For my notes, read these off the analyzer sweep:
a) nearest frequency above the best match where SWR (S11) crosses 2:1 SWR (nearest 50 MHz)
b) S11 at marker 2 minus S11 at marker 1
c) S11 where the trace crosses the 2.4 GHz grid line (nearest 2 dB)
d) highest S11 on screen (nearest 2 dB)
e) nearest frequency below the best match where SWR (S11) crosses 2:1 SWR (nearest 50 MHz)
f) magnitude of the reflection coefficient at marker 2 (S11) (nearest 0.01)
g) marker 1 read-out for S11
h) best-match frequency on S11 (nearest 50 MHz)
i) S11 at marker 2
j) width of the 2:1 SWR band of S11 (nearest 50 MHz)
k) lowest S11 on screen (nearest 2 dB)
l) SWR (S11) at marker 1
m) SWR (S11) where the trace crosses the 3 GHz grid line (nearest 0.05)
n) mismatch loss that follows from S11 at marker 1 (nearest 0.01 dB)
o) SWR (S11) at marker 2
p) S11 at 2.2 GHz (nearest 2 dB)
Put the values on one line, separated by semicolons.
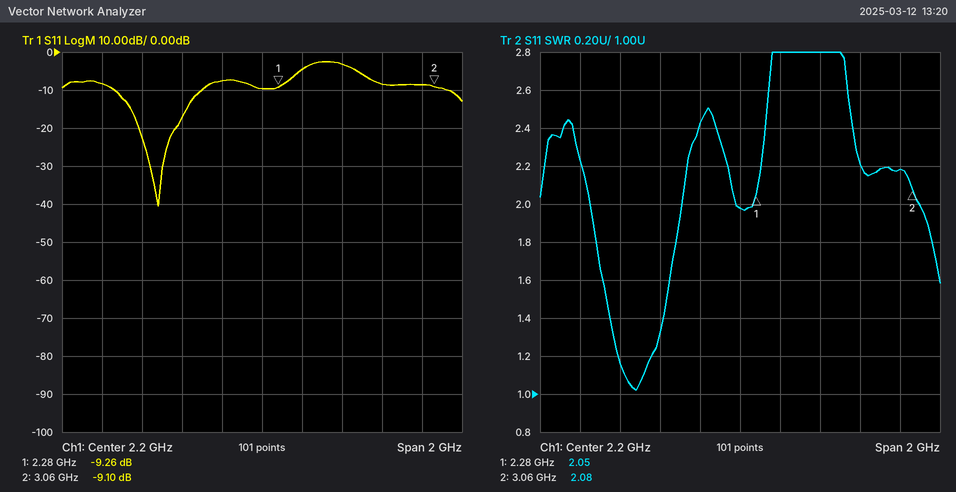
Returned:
1.90 GHz; 0.16 dB; -4 dB; -2 dB; 1.45 GHz; 0.35; -9.26 dB; 1.70 GHz; -9.10 dB; 450 MHz; -40 dB; 2.05; 2.20; 0.55 dB; 2.08; -10 dB
